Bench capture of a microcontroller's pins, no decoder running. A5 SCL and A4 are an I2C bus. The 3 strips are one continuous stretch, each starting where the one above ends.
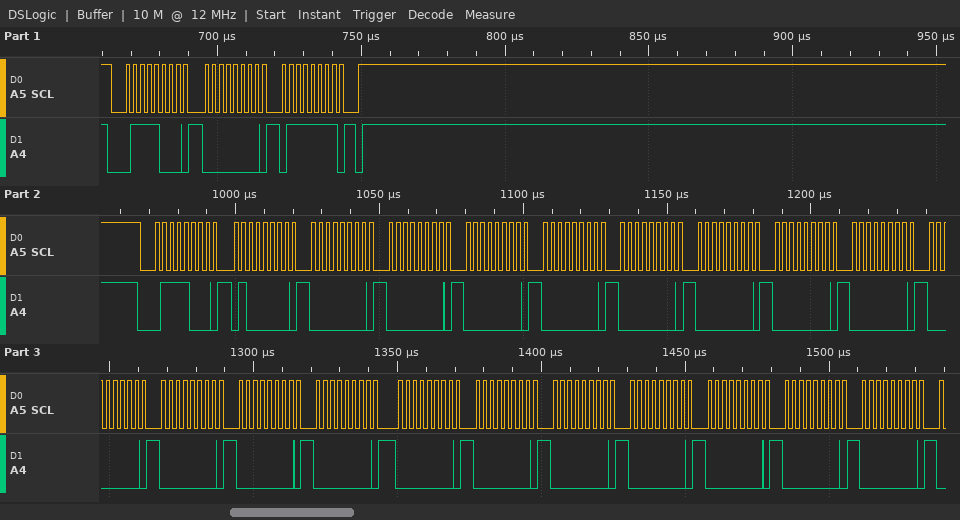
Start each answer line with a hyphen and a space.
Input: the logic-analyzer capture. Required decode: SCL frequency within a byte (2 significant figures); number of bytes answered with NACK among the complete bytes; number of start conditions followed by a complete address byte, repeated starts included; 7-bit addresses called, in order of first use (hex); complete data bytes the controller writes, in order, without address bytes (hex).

- 400 kHz
- 0
- 2
- 0x3C
- 00 7F 40 00 00 00 00 00 00 00 00 00 00 00 00 00 00 00 00 00 00 00
